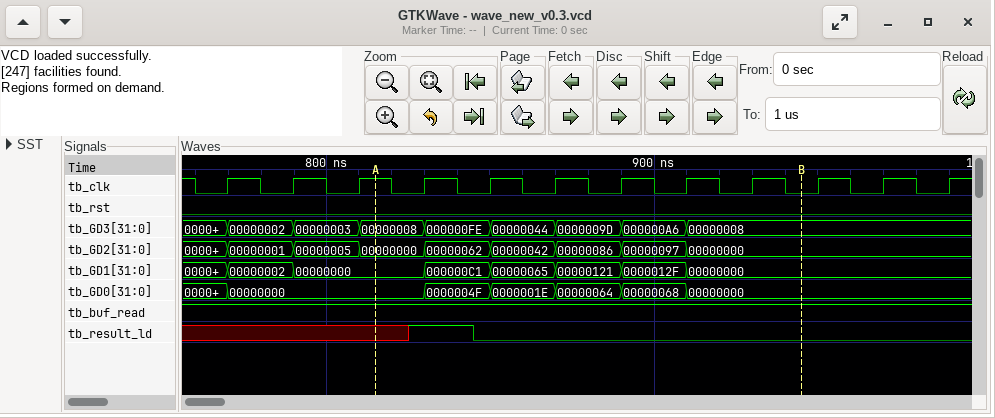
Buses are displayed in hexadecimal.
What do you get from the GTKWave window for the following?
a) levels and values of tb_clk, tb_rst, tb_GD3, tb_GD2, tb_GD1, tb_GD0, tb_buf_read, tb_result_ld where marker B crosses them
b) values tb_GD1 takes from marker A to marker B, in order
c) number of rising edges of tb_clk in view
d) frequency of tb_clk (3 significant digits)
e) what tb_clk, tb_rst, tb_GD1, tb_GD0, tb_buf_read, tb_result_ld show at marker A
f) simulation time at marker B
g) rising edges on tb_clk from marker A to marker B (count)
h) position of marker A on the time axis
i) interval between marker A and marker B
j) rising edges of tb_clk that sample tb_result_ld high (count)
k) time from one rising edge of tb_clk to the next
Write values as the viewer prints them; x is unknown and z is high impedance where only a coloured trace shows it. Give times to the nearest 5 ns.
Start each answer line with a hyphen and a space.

- tb_clk=0, tb_rst=0, tb_GD3=00000008, tb_GD2=00000000, tb_GD1=00000000, tb_GD0=00000000, tb_buf_read=1, tb_result_ld=0
- 00000000, 000000C1, 00000065, 00000121, 0000012F, 00000000
- 12
- 50.0 MHz
- tb_clk=1, tb_rst=0, tb_GD1=00000000, tb_GD0=00000000, tb_buf_read=1, tb_result_ld=x
- 945 ns
- 6
- 815 ns
- 130 ns
- 1
- 20 ns
